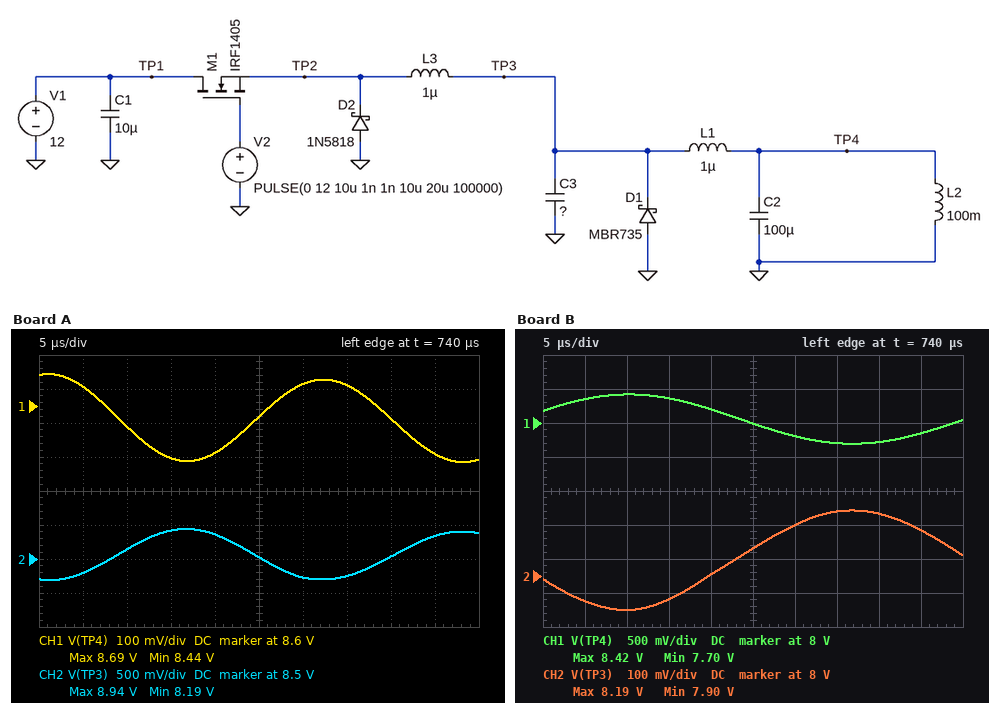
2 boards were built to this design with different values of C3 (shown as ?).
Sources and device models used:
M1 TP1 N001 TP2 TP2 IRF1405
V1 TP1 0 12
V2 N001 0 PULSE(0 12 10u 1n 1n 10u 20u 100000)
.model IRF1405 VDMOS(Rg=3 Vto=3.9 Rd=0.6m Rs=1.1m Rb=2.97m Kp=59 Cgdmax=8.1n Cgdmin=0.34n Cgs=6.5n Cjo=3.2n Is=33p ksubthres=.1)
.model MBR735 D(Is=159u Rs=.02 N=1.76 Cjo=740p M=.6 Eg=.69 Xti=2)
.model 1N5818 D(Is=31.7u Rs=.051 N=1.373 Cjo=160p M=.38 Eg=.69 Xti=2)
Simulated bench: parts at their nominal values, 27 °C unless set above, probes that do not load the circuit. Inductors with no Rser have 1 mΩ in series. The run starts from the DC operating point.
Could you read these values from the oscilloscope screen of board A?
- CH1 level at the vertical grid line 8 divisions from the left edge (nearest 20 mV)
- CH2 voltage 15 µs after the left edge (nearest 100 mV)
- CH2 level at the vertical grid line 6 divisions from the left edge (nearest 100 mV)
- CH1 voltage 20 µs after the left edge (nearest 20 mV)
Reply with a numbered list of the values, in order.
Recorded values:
1. 8.56 V
2. 8.9 V
3. 8.2 V
4. 8.46 V
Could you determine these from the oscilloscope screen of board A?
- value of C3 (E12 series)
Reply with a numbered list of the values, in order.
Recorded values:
1. 33 µF
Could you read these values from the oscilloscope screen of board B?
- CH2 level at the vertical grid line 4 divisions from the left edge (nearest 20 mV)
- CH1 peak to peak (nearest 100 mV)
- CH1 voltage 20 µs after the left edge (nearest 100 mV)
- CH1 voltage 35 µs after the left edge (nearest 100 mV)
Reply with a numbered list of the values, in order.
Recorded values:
1. 8.00 V
2. 700 mV
3. 8.2 V
4. 7.7 V
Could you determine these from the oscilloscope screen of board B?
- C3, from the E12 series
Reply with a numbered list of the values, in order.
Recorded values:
1. 270 µF
